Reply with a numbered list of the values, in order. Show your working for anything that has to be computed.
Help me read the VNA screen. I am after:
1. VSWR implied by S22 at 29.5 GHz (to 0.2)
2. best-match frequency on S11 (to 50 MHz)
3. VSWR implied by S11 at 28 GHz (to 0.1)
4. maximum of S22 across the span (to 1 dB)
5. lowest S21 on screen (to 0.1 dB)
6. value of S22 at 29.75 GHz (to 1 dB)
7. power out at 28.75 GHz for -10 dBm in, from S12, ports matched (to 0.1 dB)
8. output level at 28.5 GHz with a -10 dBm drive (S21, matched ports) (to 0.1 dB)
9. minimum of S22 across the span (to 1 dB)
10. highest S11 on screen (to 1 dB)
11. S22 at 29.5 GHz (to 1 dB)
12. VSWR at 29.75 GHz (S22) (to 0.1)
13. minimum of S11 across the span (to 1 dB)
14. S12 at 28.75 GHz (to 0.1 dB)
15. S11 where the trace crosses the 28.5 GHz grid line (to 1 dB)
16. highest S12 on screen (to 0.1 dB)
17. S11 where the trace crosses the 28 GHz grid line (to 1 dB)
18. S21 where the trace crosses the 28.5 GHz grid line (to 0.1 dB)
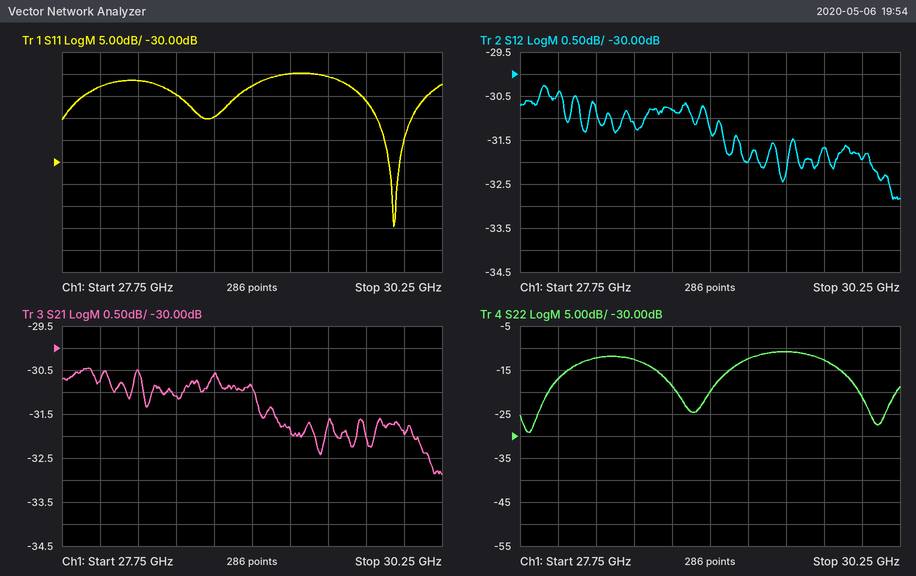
1. |Γ| = 10^(-11/20) = 0.2818; VSWR = (1 + 0.2818)/(1 − 0.2818) ≈ 1.8
2. 29.95 GHz
3. |Γ| = 10^(-13/20) = 0.2239; VSWR = (1 + 0.2239)/(1 − 0.2239) ≈ 1.6
4. -11 dB
5. -32.9 dB
6. -13 dB
7. -10 dBm + (-30.8 dB) = -40.8 dBm
8. -10 dBm + (-31.1 dB) = -41.1 dBm
9. -29 dB
10. -10 dB
11. -11 dB
12. |Γ| = 10^(-13/20) = 0.2239; VSWR = (1 + 0.2239)/(1 − 0.2239) ≈ 1.6
13. -45 dB
14. -30.8 dB
15. -15 dB
16. -30.3 dB
17. -13 dB
18. -31.1 dB
